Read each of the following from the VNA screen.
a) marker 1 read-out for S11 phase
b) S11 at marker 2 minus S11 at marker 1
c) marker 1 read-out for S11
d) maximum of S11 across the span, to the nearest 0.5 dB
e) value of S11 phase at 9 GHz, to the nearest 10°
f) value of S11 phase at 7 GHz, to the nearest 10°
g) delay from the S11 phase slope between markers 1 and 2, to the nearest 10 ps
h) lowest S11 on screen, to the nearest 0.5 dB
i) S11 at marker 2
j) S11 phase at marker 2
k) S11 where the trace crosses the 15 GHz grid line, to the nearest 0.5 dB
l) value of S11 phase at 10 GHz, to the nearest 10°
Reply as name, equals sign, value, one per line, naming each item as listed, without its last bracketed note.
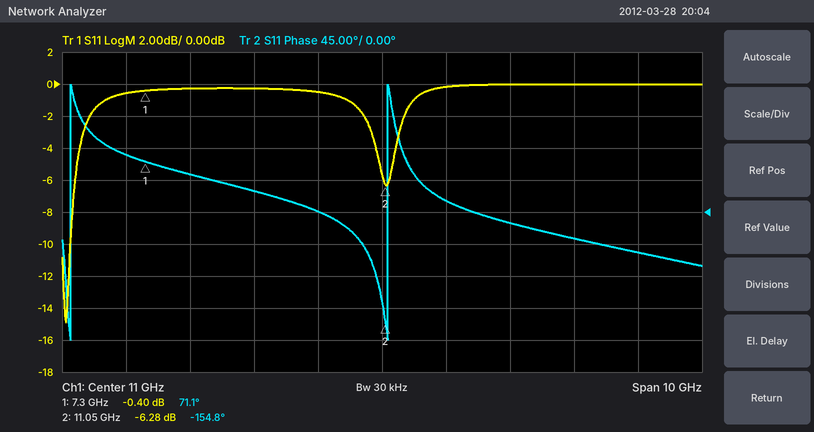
marker 1 read-out for S11 phase = 71.1°
S11 at marker 2 minus S11 at marker 1 = -5.88 dB
marker 1 read-out for S11 = -0.40 dB
maximum of S11 across the span, to the nearest 0.5 dB = 0.0 dB
value of S11 phase at 9 GHz, to the nearest 10° = 30°
value of S11 phase at 7 GHz, to the nearest 10° = 80°
delay from the S11 phase slope between markers 1 and 2, to the nearest 10 ps = 170 ps
lowest S11 on screen, to the nearest 0.5 dB = -15.0 dB
S11 at marker 2 = -6.28 dB
S11 phase at marker 2 = -154.8°
S11 where the trace crosses the 15 GHz grid line, to the nearest 0.5 dB = 0.0 dB
value of S11 phase at 10 GHz, to the nearest 10° = 0°
